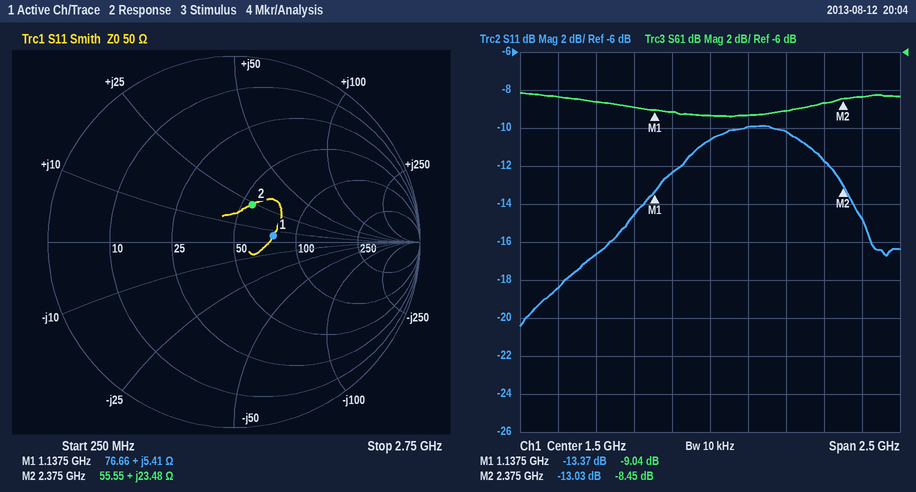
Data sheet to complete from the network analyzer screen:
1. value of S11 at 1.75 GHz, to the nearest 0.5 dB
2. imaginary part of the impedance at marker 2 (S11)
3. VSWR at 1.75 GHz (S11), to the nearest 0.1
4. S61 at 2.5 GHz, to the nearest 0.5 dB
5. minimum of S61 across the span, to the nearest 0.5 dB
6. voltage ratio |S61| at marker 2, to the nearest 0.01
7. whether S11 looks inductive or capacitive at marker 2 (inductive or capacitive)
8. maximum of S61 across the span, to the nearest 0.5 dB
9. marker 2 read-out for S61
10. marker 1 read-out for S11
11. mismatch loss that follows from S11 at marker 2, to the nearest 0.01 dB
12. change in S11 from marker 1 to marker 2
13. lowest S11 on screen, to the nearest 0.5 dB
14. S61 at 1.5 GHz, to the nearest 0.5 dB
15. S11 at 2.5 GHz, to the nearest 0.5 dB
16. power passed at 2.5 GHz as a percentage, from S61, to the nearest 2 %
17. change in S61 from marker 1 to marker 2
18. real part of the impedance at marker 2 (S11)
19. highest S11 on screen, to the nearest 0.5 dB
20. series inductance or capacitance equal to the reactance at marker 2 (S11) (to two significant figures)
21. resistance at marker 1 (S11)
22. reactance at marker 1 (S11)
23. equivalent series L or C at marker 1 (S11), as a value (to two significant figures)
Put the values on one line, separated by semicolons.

-10.0 dB; +23.48 Ω; 1.9; -8.5 dB; -9.5 dB; 0.38; inductive; -8.0 dB; -8.45 dB; -13.37 dB; 0.22 dB; 0.34 dB; -20.5 dB; -9.5 dB; -15.0 dB; 14 %; 0.59 dB; 55.55 Ω; -10.0 dB; 1.6 nH; 76.66 Ω; +5.41 Ω; 760 pH
